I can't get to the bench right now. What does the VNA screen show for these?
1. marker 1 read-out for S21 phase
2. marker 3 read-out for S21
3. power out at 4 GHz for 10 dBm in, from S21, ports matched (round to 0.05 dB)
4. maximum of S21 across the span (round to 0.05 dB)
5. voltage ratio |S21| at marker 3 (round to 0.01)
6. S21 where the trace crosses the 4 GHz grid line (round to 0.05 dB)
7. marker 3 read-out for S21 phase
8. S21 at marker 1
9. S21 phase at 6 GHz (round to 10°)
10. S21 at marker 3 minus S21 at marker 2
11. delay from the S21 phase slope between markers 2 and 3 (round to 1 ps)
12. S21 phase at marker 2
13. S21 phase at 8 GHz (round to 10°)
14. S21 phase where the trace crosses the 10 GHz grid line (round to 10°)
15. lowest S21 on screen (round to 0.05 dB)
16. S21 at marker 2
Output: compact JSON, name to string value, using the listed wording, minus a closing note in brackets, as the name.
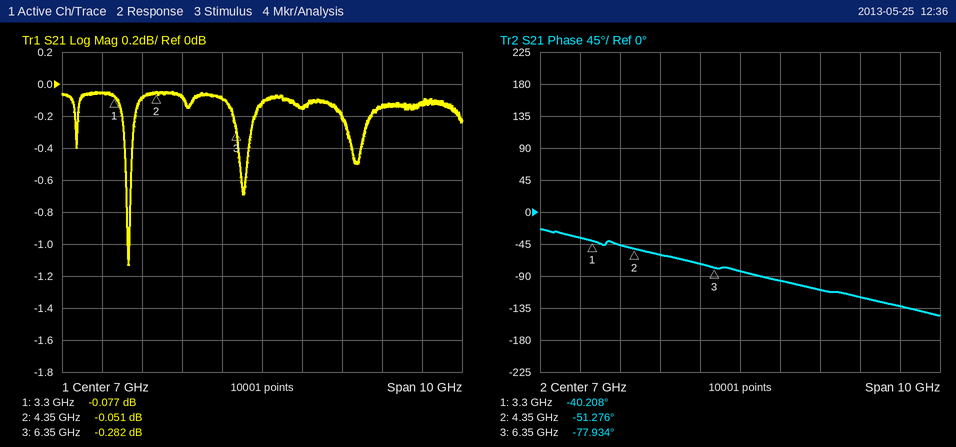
{"marker 1 read-out for S21 phase": "-40.208°", "marker 3 read-out for S21": "-0.282 dB", "power out at 4 GHz for 10 dBm in, from S21, ports matched": "9.90 dBm", "maximum of S21 across the span": "-0.05 dB", "voltage ratio |S21| at marker 3": "0.97", "S21 where the trace crosses the 4 GHz grid line": "-0.10 dB", "marker 3 read-out for S21 phase": "-77.934°", "S21 at marker 1": "-0.077 dB", "S21 phase at 6 GHz": "-70°", "S21 at marker 3 minus S21 at marker 2": "-0.231 dB", "delay from the S21 phase slope between markers 2 and 3": "37 ps", "S21 phase at marker 2": "-51.276°", "S21 phase at 8 GHz": "-100°", "S21 phase where the trace crosses the 10 GHz grid line": "-120°", "lowest S21 on screen": "-1.15 dB", "S21 at marker 2": "-0.051 dB"}
